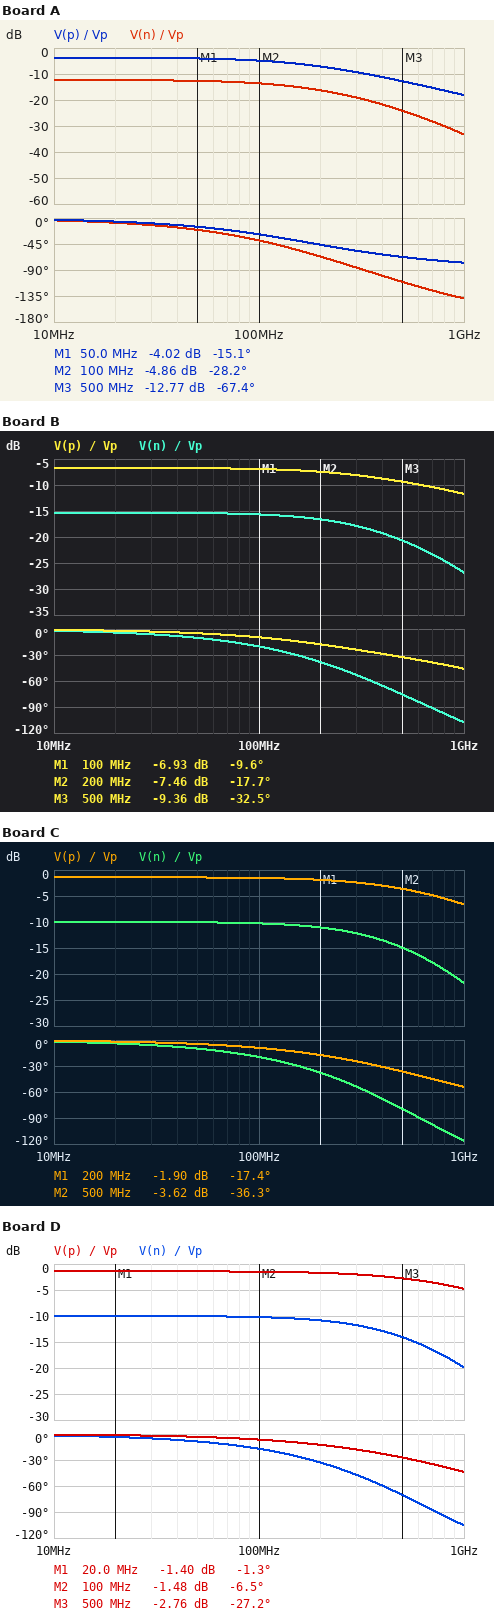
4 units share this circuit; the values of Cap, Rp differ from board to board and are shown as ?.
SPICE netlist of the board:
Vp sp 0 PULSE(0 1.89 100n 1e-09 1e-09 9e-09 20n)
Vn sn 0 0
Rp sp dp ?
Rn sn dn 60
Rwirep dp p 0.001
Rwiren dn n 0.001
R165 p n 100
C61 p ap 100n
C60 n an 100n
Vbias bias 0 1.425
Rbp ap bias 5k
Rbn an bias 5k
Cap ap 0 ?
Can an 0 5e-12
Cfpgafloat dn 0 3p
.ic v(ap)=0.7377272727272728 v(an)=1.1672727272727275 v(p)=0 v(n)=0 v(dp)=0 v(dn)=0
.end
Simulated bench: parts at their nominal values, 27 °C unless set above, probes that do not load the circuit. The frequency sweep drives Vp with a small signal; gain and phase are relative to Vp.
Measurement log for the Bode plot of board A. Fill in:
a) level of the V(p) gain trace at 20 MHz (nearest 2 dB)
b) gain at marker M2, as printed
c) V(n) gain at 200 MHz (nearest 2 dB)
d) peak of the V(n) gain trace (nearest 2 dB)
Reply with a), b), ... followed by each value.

a) -4 dB
b) -4.86 dB
c) -16 dB
d) -12 dB
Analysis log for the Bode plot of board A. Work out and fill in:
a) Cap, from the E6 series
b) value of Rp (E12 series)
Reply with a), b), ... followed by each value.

a) 15 pF
b) 82 Ω
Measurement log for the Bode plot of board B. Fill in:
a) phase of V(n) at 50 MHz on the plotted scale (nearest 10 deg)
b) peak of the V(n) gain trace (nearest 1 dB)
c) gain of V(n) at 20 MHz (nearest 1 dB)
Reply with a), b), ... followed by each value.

a) -10 deg
b) -15 dB
c) -15 dB
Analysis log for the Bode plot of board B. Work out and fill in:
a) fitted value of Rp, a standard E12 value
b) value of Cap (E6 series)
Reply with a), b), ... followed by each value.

a) 180 Ω
b) 2.2 pF
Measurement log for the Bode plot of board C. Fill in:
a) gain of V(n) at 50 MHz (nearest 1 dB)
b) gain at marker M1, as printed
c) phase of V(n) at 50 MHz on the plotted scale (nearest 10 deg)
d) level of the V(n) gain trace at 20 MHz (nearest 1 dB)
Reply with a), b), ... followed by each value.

a) -10 dB
b) -1.90 dB
c) -10 deg
d) -10 dB
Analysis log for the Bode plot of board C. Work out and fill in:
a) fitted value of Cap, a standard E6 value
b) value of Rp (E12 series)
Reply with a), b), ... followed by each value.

a) 10 pF
b) 27 Ω
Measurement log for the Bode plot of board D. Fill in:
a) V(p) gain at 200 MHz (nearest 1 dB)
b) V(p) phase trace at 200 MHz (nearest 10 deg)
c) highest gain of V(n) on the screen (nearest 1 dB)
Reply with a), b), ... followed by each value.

a) -2 dB
b) -10 deg
c) -10 dB
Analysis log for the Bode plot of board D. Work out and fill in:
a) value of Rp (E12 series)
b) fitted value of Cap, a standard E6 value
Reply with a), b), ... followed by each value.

a) 27 Ω
b) 6.8 pF
